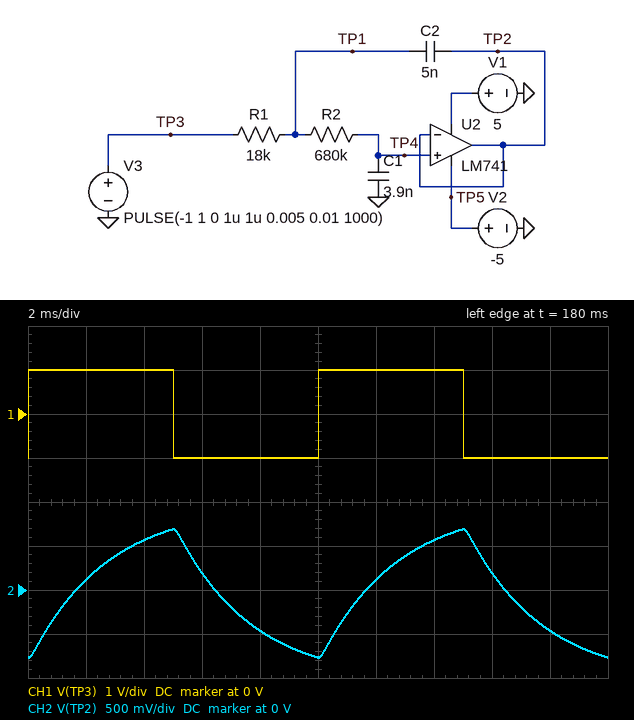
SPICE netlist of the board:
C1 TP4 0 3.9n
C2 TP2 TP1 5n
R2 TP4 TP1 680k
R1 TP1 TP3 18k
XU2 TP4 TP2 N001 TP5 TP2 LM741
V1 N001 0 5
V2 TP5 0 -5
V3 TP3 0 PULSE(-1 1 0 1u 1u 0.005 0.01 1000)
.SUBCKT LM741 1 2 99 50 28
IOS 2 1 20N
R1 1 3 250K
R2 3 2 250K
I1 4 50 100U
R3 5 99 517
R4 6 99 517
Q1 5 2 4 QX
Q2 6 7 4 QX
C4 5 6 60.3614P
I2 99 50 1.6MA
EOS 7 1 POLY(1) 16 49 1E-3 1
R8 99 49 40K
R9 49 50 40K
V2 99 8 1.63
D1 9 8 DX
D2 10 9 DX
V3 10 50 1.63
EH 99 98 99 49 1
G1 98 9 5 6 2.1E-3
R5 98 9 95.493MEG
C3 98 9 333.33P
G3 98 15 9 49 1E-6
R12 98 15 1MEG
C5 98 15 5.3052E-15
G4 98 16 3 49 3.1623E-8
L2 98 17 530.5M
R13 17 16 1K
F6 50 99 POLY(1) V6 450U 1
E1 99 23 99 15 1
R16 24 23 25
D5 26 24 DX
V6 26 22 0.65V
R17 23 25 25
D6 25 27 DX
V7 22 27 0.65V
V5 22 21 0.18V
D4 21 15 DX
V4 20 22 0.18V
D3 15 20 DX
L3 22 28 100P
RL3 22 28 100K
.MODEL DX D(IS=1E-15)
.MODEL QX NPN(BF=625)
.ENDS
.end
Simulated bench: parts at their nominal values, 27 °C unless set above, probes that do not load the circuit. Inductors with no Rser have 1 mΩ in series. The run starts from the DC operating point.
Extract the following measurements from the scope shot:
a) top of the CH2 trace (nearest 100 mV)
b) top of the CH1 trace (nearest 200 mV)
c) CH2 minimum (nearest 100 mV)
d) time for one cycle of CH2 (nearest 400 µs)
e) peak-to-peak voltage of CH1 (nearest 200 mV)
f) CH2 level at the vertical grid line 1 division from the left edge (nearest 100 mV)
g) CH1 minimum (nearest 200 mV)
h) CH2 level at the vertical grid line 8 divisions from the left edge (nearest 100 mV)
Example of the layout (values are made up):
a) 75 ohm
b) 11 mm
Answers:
a) 700 mV
b) 1.0 V
c) -800 mV
d) 10.0 ms
e) 2.0 V
f) 100 mV
g) -1.0 V
h) 200 mV
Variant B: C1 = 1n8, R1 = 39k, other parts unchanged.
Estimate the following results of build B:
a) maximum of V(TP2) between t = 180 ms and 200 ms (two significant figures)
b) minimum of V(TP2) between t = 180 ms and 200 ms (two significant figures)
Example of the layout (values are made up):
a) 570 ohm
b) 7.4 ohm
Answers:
a) 940 mV
b) -1.0 V
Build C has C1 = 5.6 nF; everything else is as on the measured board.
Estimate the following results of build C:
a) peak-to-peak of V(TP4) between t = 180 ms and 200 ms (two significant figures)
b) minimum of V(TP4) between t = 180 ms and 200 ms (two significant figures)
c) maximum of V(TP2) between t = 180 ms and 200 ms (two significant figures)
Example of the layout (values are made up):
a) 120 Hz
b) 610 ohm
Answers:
a) 1.1 V
b) -610 mV
c) 530 mV
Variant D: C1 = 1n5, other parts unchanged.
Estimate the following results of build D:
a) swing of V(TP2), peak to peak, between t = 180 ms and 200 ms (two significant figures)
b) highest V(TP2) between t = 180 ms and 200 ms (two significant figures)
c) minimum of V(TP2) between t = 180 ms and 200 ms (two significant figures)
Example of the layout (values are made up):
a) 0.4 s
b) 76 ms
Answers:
a) 2.0 V
b) 950 mV
c) -1.0 V
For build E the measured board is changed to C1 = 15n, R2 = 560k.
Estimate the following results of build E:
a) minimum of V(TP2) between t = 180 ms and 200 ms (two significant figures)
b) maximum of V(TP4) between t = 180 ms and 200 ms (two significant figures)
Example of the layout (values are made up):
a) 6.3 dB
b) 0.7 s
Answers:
a) -310 mV
b) 240 mV
